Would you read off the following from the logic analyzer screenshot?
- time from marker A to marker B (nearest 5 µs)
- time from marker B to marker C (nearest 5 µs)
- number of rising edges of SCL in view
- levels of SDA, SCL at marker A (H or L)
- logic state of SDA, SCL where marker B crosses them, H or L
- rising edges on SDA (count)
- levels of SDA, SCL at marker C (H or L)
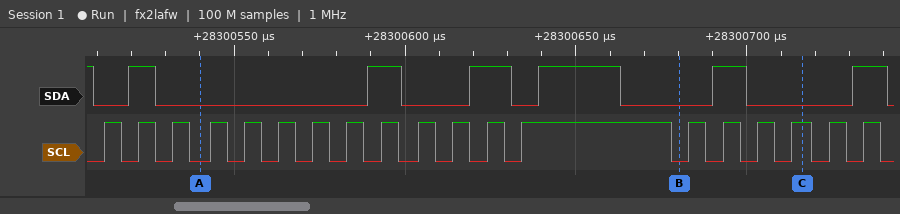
140 µs
35 µs
19
SDA=L, SCL=L
SDA=L, SCL=L
6
SDA=L, SCL=H
